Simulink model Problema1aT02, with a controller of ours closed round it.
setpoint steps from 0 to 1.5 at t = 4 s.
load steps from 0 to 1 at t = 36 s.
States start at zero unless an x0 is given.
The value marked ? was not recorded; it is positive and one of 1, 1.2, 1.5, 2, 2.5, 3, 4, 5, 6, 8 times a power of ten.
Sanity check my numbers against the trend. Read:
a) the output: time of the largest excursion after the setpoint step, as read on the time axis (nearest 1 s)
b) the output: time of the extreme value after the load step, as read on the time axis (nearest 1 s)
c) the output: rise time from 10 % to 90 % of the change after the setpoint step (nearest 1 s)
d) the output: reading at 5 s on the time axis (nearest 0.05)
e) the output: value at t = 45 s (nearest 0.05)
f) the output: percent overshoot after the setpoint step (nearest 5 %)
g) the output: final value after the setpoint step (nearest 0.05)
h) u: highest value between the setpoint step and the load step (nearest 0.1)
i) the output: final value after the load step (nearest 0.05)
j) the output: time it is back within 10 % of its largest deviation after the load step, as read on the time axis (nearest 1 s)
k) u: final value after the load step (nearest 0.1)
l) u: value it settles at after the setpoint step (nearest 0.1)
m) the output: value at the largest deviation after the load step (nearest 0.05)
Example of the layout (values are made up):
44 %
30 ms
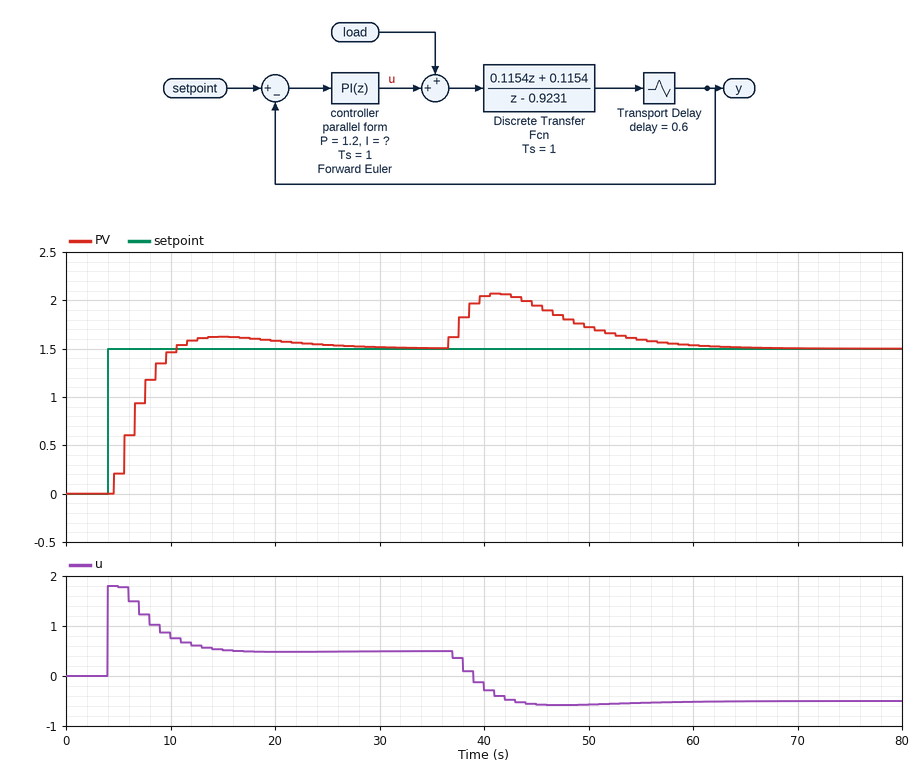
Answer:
15 s
41 s
5 s
0.20
1.95
10 %
1.50
1.8
1.50
58 s
-0.5
0.5
2.05
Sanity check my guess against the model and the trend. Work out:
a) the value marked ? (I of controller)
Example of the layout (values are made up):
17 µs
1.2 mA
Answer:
0.15
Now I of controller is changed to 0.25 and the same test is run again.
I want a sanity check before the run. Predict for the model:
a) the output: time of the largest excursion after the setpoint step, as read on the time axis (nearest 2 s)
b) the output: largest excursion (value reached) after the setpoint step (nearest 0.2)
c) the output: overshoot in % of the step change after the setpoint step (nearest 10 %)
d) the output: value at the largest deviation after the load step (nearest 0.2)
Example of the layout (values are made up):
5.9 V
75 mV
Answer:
12 s
1.8
20 %
2.0
